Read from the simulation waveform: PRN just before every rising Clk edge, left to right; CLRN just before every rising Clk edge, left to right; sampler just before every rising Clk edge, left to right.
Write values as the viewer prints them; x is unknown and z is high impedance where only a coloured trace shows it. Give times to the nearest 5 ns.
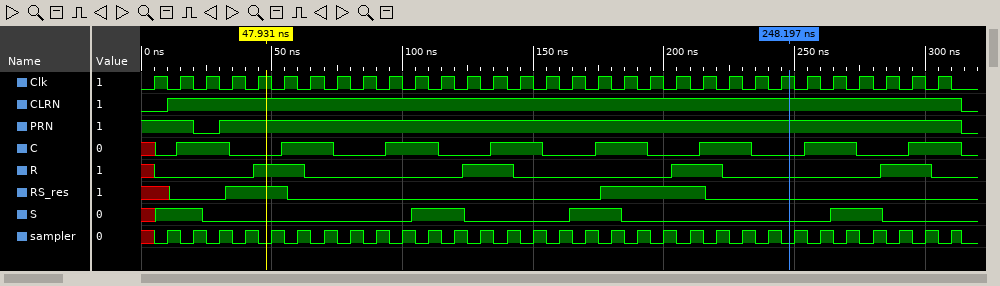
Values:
1 1 0 1 1 1 1 1 1 1 1 1 1 1 1 1 1 1 1 1 1 1 1 1 1 1 1 1 1 1 1
0 1 1 1 1 1 1 1 1 1 1 1 1 1 1 1 1 1 1 1 1 1 1 1 1 1 1 1 1 1 1
x 1 1 1 1 1 1 1 1 1 1 1 1 1 1 1 1 1 1 1 1 1 1 1 1 1 1 1 1 1 1
